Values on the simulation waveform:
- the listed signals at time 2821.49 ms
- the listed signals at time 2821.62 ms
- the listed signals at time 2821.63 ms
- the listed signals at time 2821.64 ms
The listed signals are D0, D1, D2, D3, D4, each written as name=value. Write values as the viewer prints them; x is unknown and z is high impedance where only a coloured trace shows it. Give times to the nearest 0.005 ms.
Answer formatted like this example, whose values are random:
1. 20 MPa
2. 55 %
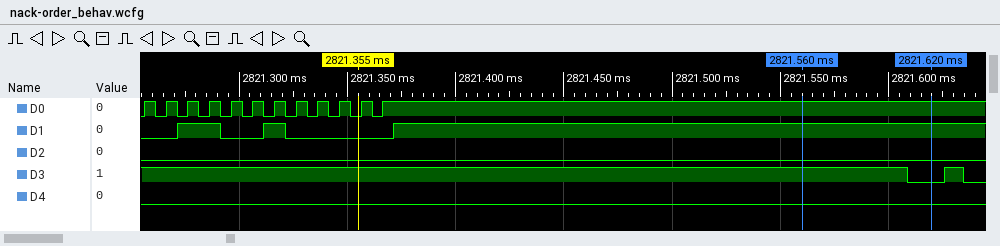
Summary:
1. D0=1, D1=1, D2=0, D3=1, D4=0
2. D0=1, D1=1, D2=0, D3=0, D4=0
3. D0=1, D1=1, D2=0, D3=1, D4=0
4. D0=1, D1=1, D2=0, D3=0, D4=0
